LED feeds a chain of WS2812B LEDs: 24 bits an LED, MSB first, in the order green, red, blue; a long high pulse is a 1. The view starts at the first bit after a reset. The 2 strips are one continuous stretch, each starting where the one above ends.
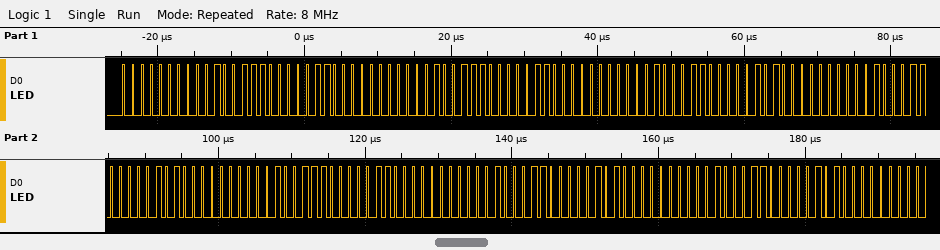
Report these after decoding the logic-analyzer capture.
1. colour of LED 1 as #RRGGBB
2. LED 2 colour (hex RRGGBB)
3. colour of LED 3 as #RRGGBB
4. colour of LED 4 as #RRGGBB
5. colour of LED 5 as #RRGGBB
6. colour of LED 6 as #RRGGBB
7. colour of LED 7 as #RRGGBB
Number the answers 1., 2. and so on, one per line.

1. #270006
2. #270006
3. #230005
4. #230005
5. #270006
6. #230005
7. #230005
